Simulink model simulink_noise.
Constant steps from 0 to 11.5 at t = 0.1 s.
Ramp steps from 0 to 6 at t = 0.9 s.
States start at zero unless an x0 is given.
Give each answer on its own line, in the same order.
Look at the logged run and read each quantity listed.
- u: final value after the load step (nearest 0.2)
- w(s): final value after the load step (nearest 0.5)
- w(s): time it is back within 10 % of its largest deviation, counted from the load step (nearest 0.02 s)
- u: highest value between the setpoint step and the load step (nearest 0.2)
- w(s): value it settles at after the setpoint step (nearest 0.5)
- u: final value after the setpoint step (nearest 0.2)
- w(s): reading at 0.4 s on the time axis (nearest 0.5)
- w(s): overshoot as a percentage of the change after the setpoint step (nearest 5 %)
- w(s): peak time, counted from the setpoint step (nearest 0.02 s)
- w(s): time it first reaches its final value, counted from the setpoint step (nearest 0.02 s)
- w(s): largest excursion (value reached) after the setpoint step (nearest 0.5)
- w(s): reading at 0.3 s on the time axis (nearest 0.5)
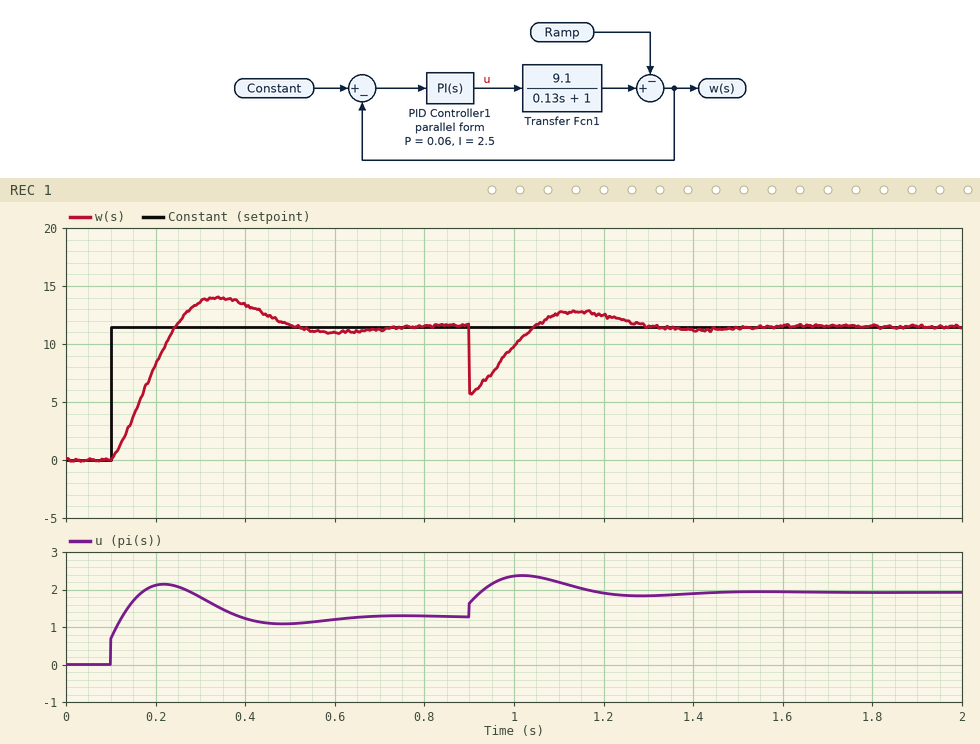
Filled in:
2.0
11.5
0.34 s
2.2
11.5
1.2
13.5
20 %
0.24 s
0.14 s
14.0
13.5
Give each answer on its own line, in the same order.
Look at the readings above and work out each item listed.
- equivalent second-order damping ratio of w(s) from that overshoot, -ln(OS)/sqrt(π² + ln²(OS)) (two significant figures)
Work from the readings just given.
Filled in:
0.46
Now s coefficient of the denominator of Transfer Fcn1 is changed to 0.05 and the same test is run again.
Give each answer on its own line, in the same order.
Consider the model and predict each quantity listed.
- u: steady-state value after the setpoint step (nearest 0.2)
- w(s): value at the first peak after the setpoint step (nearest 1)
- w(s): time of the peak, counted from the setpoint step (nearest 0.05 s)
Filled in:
1.2
12
0.20 s
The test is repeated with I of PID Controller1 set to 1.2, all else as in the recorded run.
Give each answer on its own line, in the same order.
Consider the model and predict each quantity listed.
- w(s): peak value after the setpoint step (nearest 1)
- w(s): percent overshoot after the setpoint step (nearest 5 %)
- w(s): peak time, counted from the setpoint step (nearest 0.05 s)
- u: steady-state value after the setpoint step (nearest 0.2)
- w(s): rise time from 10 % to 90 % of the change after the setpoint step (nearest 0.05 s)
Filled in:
12
10 %
0.40 s
1.2
0.20 s
